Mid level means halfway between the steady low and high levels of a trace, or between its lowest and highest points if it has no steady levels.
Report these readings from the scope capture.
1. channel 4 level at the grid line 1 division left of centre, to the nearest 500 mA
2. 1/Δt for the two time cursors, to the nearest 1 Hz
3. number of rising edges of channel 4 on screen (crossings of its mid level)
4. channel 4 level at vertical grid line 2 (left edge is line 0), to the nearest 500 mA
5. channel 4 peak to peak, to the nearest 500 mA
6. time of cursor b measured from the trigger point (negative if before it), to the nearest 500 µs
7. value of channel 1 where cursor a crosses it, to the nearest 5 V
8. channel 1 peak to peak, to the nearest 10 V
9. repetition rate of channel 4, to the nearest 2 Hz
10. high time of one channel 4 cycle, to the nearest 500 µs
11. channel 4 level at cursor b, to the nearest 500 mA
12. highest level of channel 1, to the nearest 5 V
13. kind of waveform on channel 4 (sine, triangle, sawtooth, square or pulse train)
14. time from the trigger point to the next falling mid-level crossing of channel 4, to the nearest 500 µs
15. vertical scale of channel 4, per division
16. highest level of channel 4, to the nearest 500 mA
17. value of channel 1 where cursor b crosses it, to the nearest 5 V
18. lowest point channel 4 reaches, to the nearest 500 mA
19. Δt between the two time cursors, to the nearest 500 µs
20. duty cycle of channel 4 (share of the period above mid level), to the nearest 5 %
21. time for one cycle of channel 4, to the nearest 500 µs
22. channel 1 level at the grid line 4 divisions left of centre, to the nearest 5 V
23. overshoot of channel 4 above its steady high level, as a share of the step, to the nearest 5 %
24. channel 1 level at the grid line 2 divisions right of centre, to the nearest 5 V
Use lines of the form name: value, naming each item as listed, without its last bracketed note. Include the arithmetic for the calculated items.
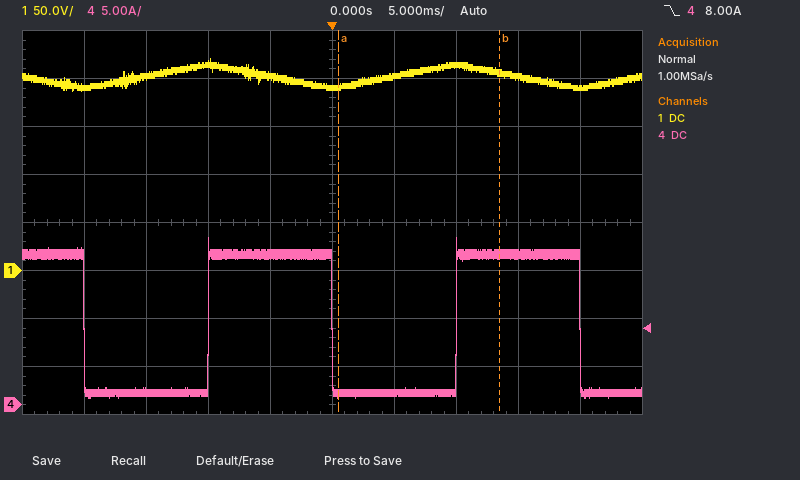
channel 4 level at the grid line 1 division left of centre, to the nearest 500 mA: 15.5 A
1/Δt for the two time cursors, to the nearest 1 Hz: 1 / 13.0 ms ≈ 77 Hz
number of rising edges of channel 4 on screen: 2
channel 4 level at vertical grid line 2 (left edge is line 0), to the nearest 500 mA: 1.5 A
channel 4 peak to peak, to the nearest 500 mA: 17.5 A − (1.0 A) = 16.5 A
time of cursor b measured from the trigger point (negative if before it), to the nearest 500 µs: +13.5 ms
value of channel 1 where cursor a crosses it, to the nearest 5 V: 190 V
channel 1 peak to peak, to the nearest 10 V: 30 V
repetition rate of channel 4, to the nearest 2 Hz: 1 / 20.0 ms ≈ 50 Hz
high time of one channel 4 cycle, to the nearest 500 µs: 10.0 ms
channel 4 level at cursor b, to the nearest 500 mA: 15.5 A
highest level of channel 1, to the nearest 5 V: 220 V
kind of waveform on channel 4: square
time from the trigger point to the next falling mid-level crossing of channel 4, to the nearest 500 µs: 20.0 ms
vertical scale of channel 4, per division: 5 A
highest level of channel 4, to the nearest 500 mA: 17.5 A
value of channel 1 where cursor b crosses it, to the nearest 5 V: 205 V
lowest point channel 4 reaches, to the nearest 500 mA: 1.0 A
Δt between the two time cursors, to the nearest 500 µs: 13.0 ms
duty cycle of channel 4 (share of the period above mid level), to the nearest 5 %: 10.0 ms / 20.0 ms ≈ 50 %
time for one cycle of channel 4, to the nearest 500 µs: 20.0 ms
channel 1 level at the grid line 4 divisions left of centre, to the nearest 5 V: 190 V
overshoot of channel 4 above its steady high level, as a share of the step, to the nearest 5 %: 10 %
channel 1 level at the grid line 2 divisions right of centre, to the nearest 5 V: 215 V
